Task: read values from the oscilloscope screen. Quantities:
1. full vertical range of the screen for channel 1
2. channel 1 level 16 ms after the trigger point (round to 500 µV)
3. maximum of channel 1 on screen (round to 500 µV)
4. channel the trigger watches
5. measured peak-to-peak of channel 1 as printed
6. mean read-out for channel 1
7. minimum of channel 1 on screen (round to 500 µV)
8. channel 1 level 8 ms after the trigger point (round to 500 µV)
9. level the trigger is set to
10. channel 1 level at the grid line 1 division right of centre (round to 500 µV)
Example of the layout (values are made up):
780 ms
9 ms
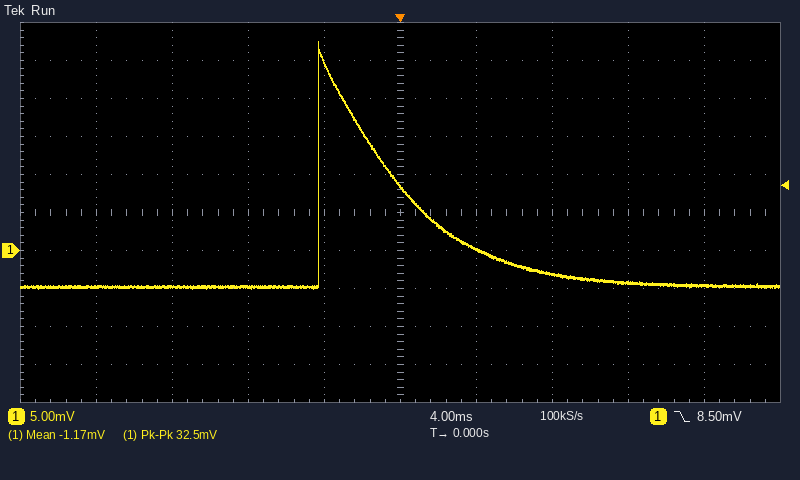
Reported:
50 mV
-4.5 mV
27.5 mV
channel 1
32.5 mV
-1.17 mV
-5.0 mV
-3.0 mV
8.50 mV
0.0 mV
